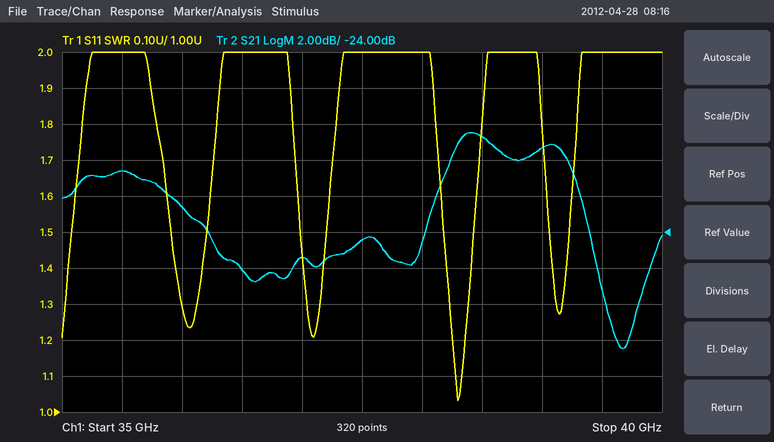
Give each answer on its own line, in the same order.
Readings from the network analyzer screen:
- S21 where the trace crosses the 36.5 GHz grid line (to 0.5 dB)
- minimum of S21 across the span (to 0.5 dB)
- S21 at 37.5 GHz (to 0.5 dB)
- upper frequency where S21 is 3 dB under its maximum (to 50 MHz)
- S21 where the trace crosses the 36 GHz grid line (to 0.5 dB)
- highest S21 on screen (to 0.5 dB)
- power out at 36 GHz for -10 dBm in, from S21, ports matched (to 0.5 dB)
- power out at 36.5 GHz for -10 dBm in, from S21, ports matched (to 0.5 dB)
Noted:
-26.0 dB
-30.5 dB
-24.5 dB
39.30 GHz
-22.5 dB
-18.5 dB
-32.5 dBm
-36.0 dBm
